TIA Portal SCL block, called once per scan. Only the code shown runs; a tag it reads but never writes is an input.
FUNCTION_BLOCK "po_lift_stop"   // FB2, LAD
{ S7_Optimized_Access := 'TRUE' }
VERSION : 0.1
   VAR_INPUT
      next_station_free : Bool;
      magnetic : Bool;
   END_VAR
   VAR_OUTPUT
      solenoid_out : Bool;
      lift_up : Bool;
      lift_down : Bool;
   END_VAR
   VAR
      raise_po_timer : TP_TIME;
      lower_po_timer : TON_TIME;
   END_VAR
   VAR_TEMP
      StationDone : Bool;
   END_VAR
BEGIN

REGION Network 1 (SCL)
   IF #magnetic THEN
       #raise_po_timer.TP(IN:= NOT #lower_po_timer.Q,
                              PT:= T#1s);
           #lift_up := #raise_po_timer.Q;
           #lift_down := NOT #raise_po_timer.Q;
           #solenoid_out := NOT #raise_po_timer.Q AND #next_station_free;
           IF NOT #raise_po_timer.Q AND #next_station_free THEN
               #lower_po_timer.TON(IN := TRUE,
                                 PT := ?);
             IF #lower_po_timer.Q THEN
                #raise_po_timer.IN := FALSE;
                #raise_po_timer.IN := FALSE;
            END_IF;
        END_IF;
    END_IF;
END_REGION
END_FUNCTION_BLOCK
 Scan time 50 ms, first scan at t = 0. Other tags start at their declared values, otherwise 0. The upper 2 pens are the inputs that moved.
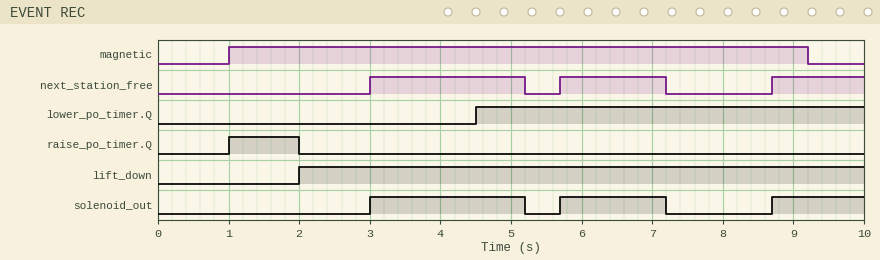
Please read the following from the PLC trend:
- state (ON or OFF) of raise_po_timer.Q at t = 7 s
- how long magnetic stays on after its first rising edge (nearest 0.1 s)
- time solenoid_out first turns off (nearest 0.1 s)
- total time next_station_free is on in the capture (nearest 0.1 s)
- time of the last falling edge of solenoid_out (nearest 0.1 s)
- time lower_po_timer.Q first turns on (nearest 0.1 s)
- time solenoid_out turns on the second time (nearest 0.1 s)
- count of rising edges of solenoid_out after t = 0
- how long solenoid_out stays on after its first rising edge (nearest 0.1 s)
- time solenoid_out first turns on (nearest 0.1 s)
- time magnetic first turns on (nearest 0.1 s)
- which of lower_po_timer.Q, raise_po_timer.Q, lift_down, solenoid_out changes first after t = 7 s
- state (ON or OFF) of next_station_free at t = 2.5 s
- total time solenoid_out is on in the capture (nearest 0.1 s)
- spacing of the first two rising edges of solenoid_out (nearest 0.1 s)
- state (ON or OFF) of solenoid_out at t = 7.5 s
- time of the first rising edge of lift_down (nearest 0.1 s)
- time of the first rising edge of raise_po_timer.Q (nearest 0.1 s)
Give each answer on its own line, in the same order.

OFF
8.2 s
5.2 s
5.0 s
7.2 s
4.5 s
5.7 s
3
2.2 s
3.0 s
1.0 s
solenoid_out
OFF
5.0 s
2.7 s
OFF
2.0 s
1.0 s
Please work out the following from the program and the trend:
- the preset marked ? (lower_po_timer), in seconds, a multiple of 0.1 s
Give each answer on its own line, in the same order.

1.5 s
